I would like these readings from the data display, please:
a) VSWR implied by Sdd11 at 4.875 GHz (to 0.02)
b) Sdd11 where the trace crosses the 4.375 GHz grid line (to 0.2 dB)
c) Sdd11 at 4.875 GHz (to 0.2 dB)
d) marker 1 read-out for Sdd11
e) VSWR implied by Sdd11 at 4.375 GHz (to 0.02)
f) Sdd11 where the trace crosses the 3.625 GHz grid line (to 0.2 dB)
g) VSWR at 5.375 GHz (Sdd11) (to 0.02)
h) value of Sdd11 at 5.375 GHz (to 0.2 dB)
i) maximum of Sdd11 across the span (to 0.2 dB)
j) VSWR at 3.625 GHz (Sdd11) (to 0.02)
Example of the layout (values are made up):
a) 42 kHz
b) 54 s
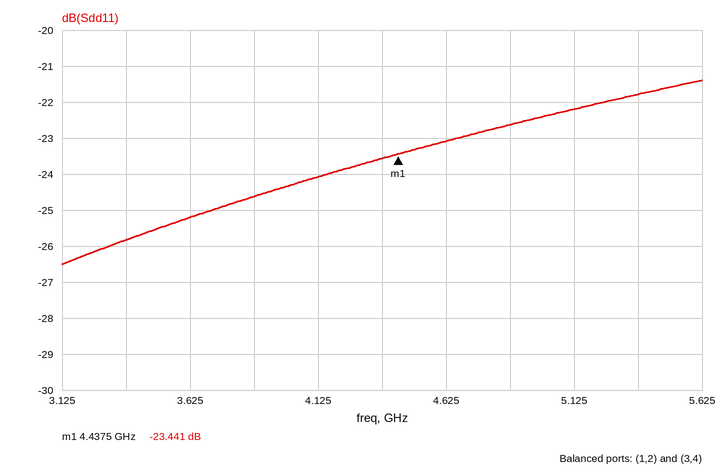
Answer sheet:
a) 1.16
b) -23.6 dB
c) -22.6 dB
d) -23.441 dB
e) 1.14
f) -25.2 dB
g) 1.18
h) -21.8 dB
i) -21.4 dB
j) 1.12
